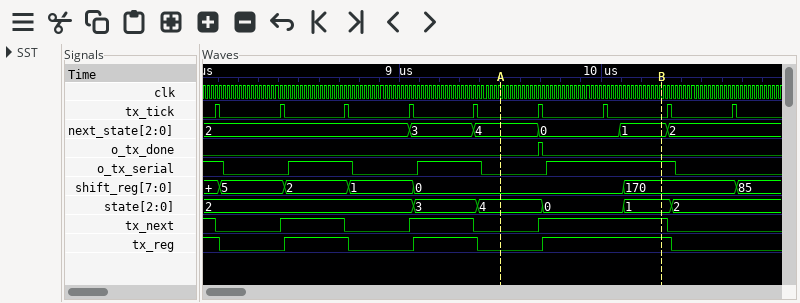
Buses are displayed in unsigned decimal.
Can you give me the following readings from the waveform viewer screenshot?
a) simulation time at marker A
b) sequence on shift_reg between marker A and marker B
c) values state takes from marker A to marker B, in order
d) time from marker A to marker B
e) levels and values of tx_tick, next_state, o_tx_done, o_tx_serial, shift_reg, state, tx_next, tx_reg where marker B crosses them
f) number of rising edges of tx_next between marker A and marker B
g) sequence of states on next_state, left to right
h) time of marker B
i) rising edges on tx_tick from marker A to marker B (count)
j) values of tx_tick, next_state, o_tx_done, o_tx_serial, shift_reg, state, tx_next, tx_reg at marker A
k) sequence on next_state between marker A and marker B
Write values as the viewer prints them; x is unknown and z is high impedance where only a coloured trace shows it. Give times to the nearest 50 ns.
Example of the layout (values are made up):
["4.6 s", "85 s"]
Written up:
["9500 ns", "0, 170", "4, 0, 1", "800 ns", "tx_tick=0, next_state=1, o_tx_done=0, o_tx_serial=1, shift_reg=170, state=1, tx_next=1, tx_reg=1", "1", "2, 3, 4, 0, 1, 2", "10300 ns", "2", "tx_tick=0, next_state=4, o_tx_done=0, o_tx_serial=0, shift_reg=0, state=4, tx_next=0, tx_reg=0", "4, 0, 1"]
